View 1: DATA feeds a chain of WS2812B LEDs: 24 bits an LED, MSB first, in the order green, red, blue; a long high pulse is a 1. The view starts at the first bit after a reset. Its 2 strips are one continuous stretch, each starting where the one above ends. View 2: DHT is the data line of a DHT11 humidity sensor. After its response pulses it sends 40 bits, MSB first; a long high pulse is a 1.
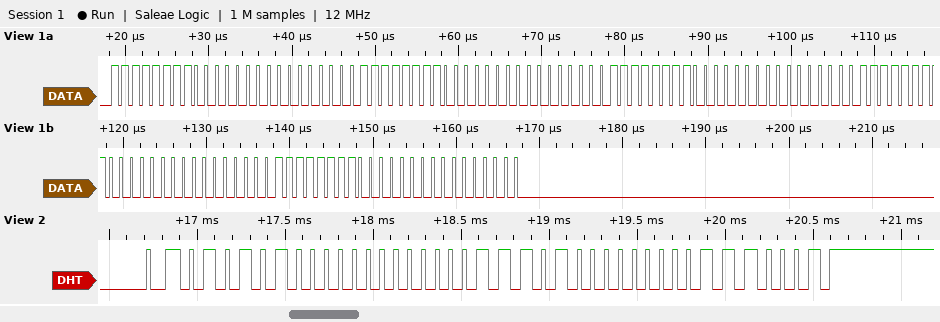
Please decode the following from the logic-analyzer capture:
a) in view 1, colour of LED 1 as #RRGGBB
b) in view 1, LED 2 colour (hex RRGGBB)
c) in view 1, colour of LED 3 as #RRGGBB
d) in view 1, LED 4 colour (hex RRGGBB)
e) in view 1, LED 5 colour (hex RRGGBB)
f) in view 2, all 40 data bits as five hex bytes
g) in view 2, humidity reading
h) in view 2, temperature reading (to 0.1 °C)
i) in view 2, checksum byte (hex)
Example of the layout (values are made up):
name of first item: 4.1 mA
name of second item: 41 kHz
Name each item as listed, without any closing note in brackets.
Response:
in view 1, colour of LED 1 as #RRGGBB: #00FF00
in view 1, LED 2 colour: #00FF00
in view 1, colour of LED 3 as #RRGGBB: #00FF00
in view 1, LED 4 colour: #00FF00
in view 1, LED 5 colour: #00FF00
in view 2, all 40 data bits as five hex bytes: 54 00 1D 00 71
in view 2, humidity reading: 84 %
in view 2, temperature reading: 29.0 °C
in view 2, checksum byte: 0x71
